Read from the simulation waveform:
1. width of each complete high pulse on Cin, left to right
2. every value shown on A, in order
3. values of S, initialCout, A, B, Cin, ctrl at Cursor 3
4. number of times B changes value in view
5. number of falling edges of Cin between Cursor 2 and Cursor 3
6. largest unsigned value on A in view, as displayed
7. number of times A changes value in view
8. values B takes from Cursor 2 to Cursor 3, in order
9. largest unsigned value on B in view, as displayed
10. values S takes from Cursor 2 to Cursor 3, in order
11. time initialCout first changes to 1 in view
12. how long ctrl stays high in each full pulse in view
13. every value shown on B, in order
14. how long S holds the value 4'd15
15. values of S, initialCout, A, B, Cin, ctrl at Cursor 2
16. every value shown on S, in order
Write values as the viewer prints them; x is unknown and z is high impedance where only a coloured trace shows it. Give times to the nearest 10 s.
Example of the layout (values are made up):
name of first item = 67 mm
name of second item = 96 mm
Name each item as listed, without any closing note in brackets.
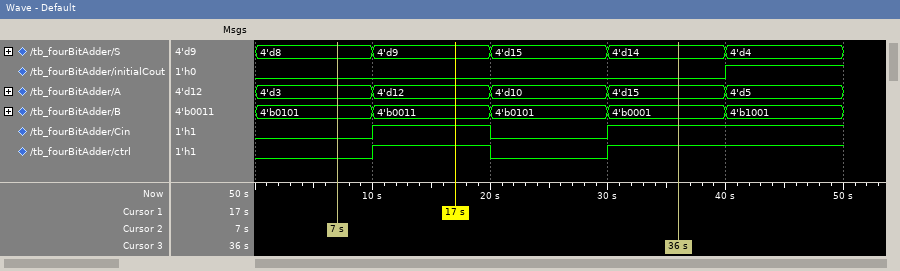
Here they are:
width of each complete high pulse on Cin, left to right = 10 s
every value shown on A, in order = 4'd3, 4'd12, 4'd10, 4'd15, 4'd5
values of S, initialCout, A, B, Cin, ctrl at Cursor 3 = S=4'd14, initialCout=0, A=4'd15, B=4'b0001, Cin=1, ctrl=1
number of times B changes value in view = 4
number of falling edges of Cin between Cursor 2 and Cursor 3 = 1
largest unsigned value on A in view, as displayed = 4'd15
number of times A changes value in view = 4
values B takes from Cursor 2 to Cursor 3, in order = 4'b0101, 4'b0011, 4'b0101, 4'b0001
largest unsigned value on B in view, as displayed = 4'b1001
values S takes from Cursor 2 to Cursor 3, in order = 4'd8, 4'd9, 4'd15, 4'd14
time initialCout first changes to 1 in view = 40 s
how long ctrl stays high in each full pulse in view = 10 s
every value shown on B, in order = 4'b0101, 4'b0011, 4'b0101, 4'b0001, 4'b1001
how long S holds the value 4'd15 = 10 s
values of S, initialCout, A, B, Cin, ctrl at Cursor 2 = S=4'd8, initialCout=0, A=4'd3, B=4'b0101, Cin=0, ctrl=0
every value shown on S, in order = 4'd8, 4'd9, 4'd15, 4'd14, 4'd4
